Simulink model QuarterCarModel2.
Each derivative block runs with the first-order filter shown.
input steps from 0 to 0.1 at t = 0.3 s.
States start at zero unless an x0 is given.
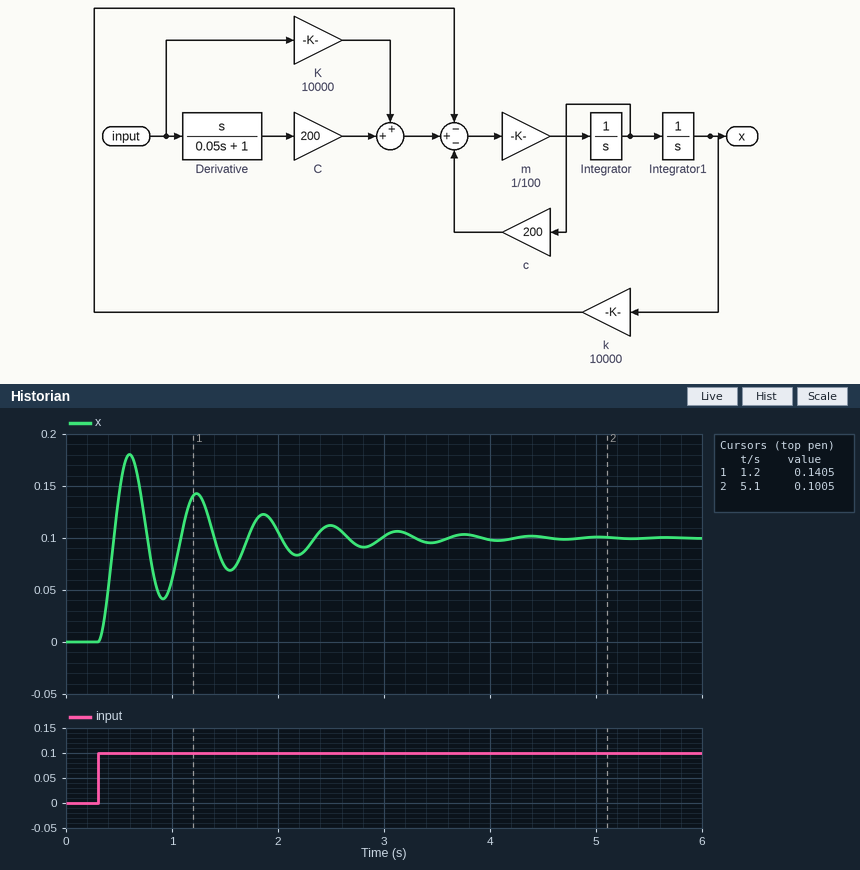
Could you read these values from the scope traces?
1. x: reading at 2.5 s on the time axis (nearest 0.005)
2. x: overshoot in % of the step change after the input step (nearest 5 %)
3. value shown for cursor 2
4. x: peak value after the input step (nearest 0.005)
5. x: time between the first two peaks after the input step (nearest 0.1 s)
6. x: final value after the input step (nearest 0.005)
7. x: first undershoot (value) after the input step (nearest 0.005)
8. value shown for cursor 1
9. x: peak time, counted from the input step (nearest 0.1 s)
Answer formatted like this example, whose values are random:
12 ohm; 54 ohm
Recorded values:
0.110; 80 %; 0.1005; 0.180; 0.6 s; 0.100; 0.040; 0.1405; 0.3 s
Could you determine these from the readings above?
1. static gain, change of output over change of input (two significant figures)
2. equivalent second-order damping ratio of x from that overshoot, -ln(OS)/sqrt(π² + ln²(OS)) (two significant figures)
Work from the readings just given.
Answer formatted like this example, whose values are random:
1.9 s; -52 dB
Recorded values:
1.0; 0.071
